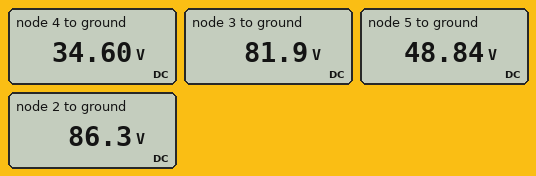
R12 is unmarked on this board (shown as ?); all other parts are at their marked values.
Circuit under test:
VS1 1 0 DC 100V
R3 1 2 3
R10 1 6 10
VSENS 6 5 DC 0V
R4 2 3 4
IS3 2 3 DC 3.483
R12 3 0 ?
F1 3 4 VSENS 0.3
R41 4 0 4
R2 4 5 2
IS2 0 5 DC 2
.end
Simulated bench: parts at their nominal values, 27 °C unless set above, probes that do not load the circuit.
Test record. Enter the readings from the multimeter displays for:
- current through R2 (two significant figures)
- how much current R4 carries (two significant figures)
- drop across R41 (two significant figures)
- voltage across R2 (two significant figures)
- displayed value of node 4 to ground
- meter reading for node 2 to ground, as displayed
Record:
7.1 A
1.1 A
35 V
14 V
34.60 V
86.3 V
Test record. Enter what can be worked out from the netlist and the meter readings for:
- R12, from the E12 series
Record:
27 Ω
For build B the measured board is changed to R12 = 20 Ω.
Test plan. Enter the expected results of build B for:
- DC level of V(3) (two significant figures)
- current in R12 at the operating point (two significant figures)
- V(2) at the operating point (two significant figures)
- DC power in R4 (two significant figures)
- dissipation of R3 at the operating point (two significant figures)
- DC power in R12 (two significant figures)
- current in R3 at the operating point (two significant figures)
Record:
76 V
3.8 A
84 V
14 W
86 W
290 W
5.4 A
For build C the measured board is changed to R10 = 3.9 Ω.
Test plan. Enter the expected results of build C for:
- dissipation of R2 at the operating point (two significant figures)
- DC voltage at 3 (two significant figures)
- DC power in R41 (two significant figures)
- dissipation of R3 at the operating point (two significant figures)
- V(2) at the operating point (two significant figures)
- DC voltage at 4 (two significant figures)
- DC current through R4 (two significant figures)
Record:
200 W
77 V
610 W
82 W
84 V
49 V
1.8 A
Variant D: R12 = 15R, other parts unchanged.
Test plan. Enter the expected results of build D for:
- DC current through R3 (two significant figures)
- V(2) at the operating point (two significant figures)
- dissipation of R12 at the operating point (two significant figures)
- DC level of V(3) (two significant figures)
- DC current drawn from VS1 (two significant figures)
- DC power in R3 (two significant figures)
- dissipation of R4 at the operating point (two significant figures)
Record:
6.2 A
81 V
330 W
70 V
11 A
120 W
30 W
